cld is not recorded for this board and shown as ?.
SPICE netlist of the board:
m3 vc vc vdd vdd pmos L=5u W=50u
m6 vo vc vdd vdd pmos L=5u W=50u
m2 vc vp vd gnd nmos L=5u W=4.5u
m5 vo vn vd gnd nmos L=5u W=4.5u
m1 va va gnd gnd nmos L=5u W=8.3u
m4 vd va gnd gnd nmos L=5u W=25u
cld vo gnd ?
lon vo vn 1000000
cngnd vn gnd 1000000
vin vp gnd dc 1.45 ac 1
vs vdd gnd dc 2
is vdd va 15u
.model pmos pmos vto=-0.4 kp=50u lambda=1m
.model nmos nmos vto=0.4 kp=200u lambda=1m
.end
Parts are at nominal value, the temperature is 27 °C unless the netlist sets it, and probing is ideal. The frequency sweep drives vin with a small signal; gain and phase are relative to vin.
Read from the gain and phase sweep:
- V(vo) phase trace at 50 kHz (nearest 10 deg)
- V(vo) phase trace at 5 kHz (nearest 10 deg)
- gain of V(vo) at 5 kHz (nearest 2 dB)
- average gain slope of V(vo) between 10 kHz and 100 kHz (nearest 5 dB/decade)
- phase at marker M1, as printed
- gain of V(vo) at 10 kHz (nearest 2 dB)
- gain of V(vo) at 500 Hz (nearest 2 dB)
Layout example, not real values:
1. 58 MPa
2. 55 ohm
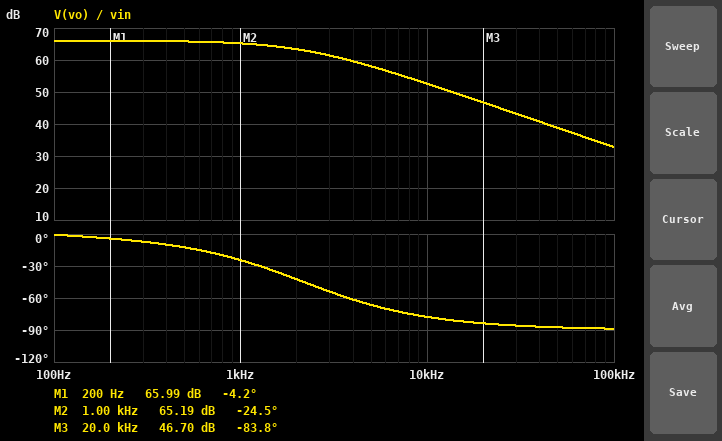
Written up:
1. -90 deg
2. -70 deg
3. 58 dB
4. -20 dB/decade
5. -4.2 deg
6. 52 dB
7. 66 dB
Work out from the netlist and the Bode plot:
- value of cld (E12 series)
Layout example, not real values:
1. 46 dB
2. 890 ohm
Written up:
1. 3.3 pF
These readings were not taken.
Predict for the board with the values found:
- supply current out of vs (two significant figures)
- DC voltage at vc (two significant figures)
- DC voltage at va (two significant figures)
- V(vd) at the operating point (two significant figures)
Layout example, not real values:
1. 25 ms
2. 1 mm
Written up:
1. 60 µA
2. 1.3 V
3. 700 mV
4. 550 mV
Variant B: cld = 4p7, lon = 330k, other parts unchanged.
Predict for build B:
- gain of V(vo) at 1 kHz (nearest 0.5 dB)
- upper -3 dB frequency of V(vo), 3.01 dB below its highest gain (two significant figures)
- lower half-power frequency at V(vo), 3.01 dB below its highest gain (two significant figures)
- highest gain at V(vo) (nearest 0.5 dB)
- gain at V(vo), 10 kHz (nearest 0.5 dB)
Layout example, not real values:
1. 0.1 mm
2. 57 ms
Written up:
1. 64.5 dB
2. 1.5 kHz
3. 11 Hz
4. 66.0 dB
5. 49.5 dB
